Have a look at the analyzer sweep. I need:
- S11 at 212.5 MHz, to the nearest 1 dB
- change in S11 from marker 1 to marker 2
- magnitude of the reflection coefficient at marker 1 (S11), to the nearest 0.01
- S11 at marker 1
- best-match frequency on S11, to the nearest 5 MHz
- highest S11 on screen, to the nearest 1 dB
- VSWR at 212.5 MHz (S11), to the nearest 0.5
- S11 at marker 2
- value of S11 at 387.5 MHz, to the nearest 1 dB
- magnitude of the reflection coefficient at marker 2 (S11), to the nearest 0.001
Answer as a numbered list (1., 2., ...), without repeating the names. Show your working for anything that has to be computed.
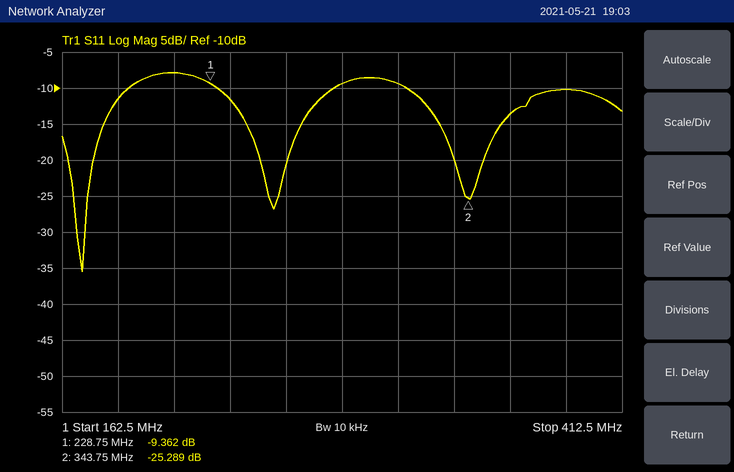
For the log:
1. -8 dB
2. -25.289 − (-9.362) = -15.927 dB
3. 10^(-9.362/20) ≈ 0.34
4. -9.362 dB
5. 170 MHz
6. -8 dB
7. |Γ| = 10^(-8/20) = 0.3981; VSWR = (1 + 0.3981)/(1 − 0.3981) ≈ 2.32, so 2.5 to the nearest 0.5
8. -25.289 dB
9. -10 dB
10. 10^(-25.289/20) ≈ 0.054
